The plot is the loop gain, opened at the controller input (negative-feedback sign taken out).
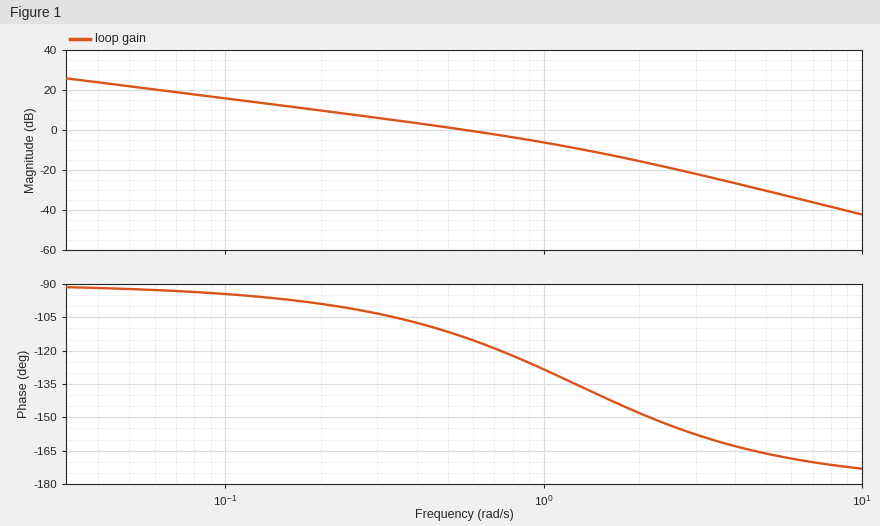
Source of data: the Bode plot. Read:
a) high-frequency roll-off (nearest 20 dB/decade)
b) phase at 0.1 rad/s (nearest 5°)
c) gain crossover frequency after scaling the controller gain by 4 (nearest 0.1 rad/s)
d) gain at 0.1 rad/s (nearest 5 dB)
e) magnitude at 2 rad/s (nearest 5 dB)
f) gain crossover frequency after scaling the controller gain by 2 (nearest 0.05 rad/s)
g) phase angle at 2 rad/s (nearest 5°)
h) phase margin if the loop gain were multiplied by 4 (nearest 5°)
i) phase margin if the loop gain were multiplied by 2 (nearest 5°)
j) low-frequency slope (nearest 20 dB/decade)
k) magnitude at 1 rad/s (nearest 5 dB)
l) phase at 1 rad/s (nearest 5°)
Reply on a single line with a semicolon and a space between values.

-40 dB/decade; -95°; 1.6 rad/s; 15 dB; -15 dB; 1.00 rad/s; -150°; 40°; 50°; -20 dB/decade; -5 dB; -130°
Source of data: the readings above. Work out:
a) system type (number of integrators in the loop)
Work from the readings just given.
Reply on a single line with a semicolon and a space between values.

1
